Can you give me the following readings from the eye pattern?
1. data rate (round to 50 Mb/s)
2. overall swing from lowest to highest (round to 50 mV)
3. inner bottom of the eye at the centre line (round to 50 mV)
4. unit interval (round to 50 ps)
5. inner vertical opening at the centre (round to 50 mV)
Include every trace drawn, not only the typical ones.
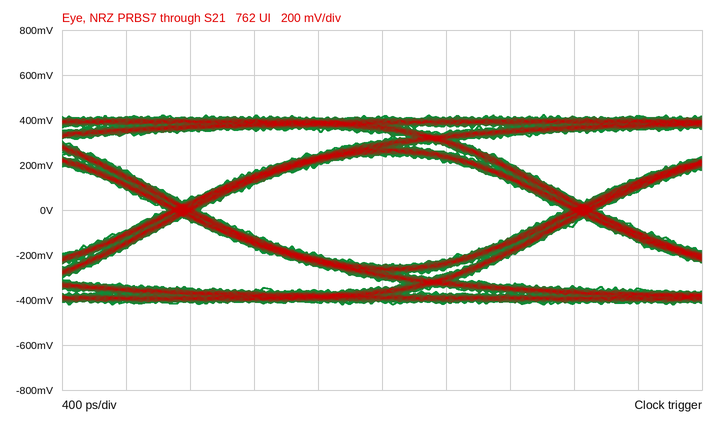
400 Mb/s
850 mV
-250 mV
2.50 ns
500 mV
